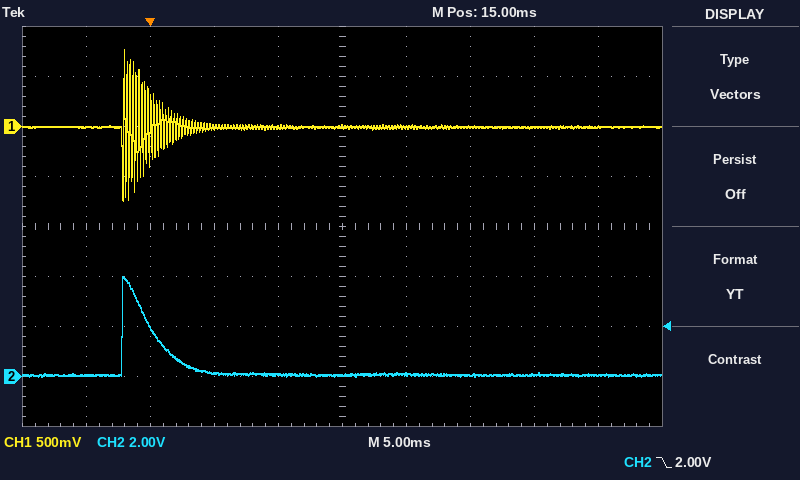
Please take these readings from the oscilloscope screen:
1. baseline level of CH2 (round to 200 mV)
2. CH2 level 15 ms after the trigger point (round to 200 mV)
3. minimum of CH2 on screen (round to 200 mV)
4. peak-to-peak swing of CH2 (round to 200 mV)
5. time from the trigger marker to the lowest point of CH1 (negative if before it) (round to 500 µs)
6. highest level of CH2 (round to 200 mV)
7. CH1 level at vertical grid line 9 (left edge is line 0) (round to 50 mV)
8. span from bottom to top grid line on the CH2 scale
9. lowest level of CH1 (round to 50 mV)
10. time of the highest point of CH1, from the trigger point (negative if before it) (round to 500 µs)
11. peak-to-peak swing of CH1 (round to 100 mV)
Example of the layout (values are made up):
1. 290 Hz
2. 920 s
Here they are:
1. 0.0 V
2. 0.0 V
3. 0.0 V
4. 4.0 V
5. -2.0 ms
6. 4.0 V
7. 0 mV
8. 16 V
9. -750 mV
10. -2.0 ms
11. 1.50 V
